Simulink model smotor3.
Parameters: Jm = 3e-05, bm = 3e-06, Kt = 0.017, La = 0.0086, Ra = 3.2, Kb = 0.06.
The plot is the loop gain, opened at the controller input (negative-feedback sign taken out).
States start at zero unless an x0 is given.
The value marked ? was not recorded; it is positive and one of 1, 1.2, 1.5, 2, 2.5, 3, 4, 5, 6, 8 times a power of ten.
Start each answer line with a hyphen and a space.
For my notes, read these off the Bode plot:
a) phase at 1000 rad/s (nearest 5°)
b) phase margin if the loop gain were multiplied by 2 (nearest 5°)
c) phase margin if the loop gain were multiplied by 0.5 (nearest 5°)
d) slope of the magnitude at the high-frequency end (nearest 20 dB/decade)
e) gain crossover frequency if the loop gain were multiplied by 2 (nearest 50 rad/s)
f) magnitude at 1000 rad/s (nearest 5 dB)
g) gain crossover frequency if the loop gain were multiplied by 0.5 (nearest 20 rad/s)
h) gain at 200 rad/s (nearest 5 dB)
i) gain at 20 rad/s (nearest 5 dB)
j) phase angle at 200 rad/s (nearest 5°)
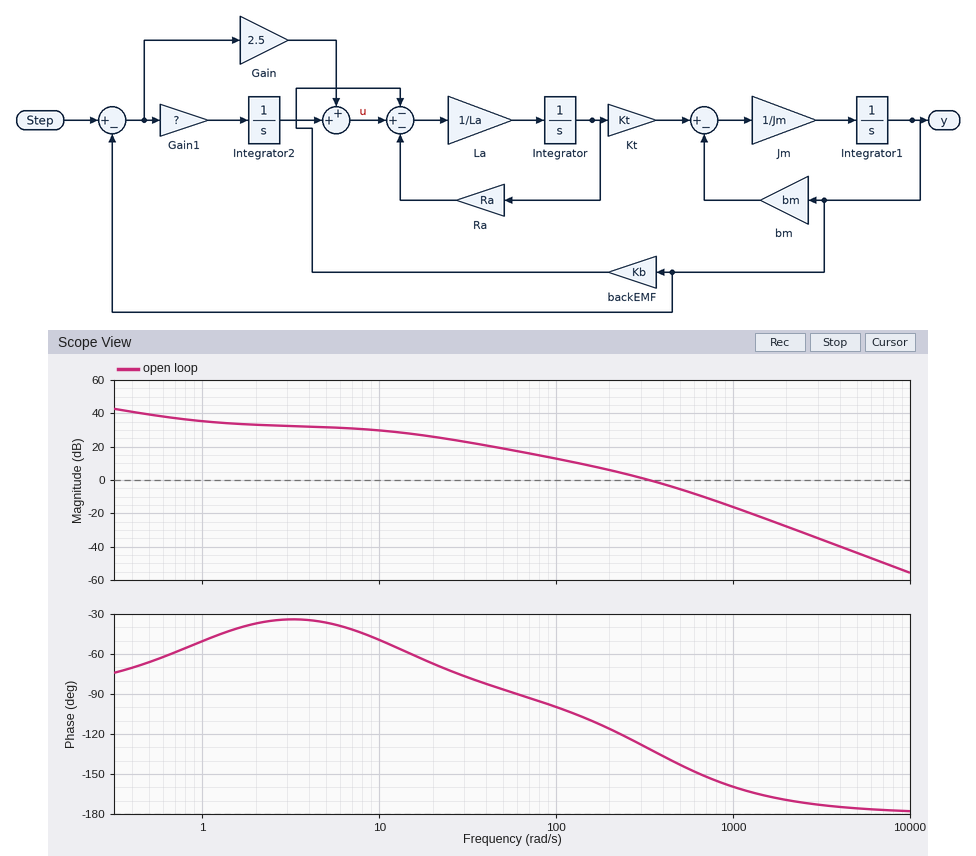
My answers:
- -160°
- 35°
- 65°
- -40 dB/decade
- 500 rad/s
- -15 dB
- 200 rad/s
- 5 dB
- 25 dB
- -115°
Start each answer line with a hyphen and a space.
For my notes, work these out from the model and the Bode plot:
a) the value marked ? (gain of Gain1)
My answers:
- 2.5
